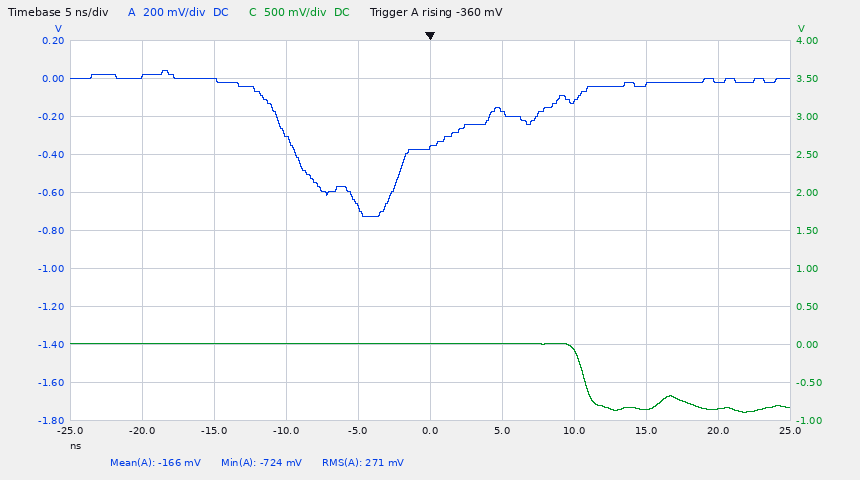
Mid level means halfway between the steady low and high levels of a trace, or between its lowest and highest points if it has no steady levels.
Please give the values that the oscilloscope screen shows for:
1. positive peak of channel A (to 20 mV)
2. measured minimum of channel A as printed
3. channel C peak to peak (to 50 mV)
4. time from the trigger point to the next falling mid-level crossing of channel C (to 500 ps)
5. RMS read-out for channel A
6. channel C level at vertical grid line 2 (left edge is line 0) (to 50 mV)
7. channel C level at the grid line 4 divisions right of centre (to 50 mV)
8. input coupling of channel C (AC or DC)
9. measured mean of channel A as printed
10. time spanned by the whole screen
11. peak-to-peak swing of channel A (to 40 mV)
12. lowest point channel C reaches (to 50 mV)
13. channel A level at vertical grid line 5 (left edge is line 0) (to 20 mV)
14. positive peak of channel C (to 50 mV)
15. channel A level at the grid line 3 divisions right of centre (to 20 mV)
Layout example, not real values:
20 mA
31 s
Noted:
40 mV
-724 mV
900 mV
10.5 ns
271 mV
0 mV
-850 mV
DC
-166 mV
50 ns
760 mV
-900 mV
-360 mV
0 mV
-40 mV
